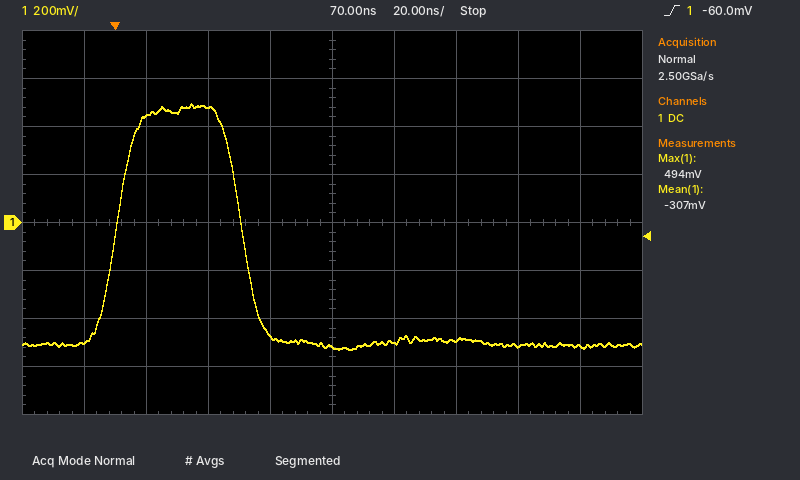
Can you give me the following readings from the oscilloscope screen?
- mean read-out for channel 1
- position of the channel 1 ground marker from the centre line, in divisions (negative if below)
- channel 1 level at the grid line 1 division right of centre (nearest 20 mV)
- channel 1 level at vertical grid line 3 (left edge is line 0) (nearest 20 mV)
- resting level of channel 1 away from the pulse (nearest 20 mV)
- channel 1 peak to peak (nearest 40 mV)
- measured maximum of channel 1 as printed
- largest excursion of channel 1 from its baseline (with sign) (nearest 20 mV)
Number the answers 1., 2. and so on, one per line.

1. -307 mV
2. 0.0 div
3. -500 mV
4. 480 mV
5. -500 mV
6. 1.04 V
7. 494 mV
8. +1.00 V
